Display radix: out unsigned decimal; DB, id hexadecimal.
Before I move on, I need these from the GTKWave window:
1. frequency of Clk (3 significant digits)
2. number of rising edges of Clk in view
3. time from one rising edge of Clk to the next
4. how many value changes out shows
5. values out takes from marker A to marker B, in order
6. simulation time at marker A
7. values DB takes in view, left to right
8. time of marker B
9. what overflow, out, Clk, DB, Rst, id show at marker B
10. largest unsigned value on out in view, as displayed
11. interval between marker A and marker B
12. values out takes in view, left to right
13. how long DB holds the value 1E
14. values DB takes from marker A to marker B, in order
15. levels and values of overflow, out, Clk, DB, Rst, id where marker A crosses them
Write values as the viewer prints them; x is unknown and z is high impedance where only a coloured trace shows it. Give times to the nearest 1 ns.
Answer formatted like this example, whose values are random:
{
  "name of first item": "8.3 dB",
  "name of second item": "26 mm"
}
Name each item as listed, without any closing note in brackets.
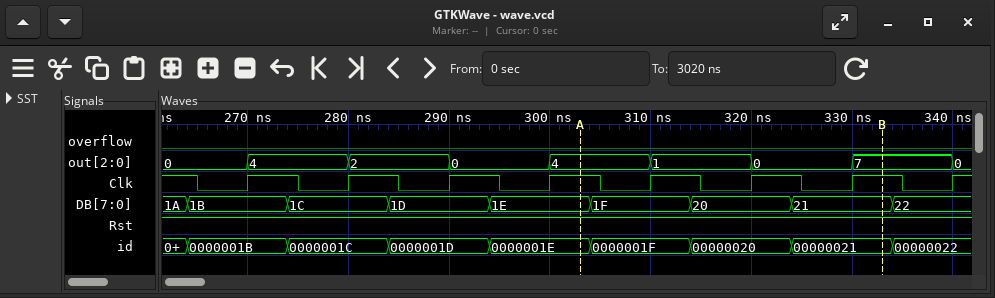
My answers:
{
  "frequency of Clk": "100 MHz",
  "number of rising edges of Clk in view": "8",
  "time from one rising edge of Clk to the next": "10 ns",
  "how many value changes out shows": "8",
  "values out takes from marker A to marker B, in order": "4, 1, 0, 7",
  "simulation time at marker A": "303 ns",
  "values DB takes in view, left to right": "1A, 1B, 1C, 1D, 1E, 1F, 20, 21, 22",
  "time of marker B": "333 ns",
  "what overflow, out, Clk, DB, Rst, id show at marker B": "overflow=0, out=7, Clk=1, DB=21, Rst=1, id=00000021",
  "largest unsigned value on out in view, as displayed": "7",
  "interval between marker A and marker B": "30 ns",
  "values out takes in view, left to right": "0, 4, 2, 0, 4, 1, 0, 7, 0",
  "how long DB holds the value 1E": "10 ns",
  "values DB takes from marker A to marker B, in order": "1E, 1F, 20, 21",
  "levels and values of overflow, out, Clk, DB, Rst, id where marker A crosses them": "overflow=0, out=4, Clk=1, DB=1E, Rst=1, id=0000001E"
}
